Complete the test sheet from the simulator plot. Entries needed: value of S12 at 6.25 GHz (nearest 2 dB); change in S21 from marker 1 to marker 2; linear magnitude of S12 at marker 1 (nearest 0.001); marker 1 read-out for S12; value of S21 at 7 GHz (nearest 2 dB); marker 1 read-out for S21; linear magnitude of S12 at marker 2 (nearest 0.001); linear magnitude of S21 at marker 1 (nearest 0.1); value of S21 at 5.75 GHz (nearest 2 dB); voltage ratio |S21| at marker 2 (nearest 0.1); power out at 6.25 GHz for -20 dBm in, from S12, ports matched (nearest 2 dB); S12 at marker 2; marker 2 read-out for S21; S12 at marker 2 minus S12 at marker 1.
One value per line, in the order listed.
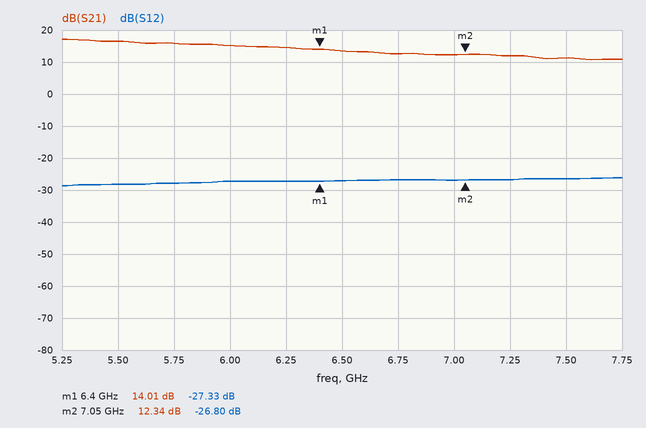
-28 dB
-1.67 dB
0.043
-27.33 dB
12 dB
14.01 dB
0.046
5.0
16 dB
4.1
-48 dBm
-26.80 dB
12.34 dB
0.53 dB
